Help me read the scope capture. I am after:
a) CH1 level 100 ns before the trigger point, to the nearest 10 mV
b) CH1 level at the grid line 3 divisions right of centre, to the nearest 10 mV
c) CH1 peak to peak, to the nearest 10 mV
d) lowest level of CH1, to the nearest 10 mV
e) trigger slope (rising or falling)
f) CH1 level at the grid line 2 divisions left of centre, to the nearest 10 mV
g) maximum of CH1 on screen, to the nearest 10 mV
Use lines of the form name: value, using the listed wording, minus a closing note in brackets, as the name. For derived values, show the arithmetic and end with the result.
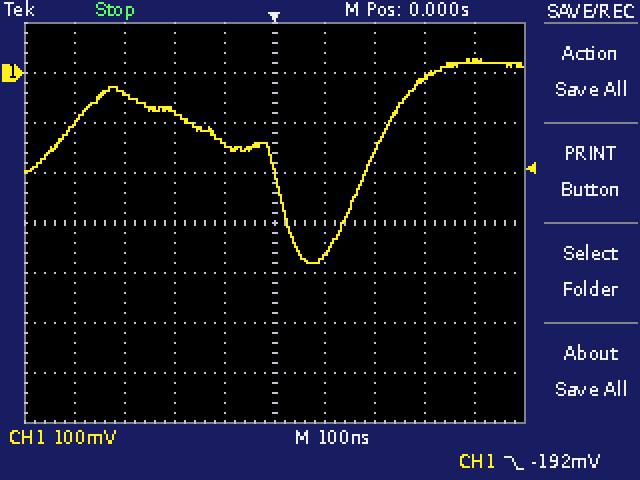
CH1 level 100 ns before the trigger point, to the nearest 10 mV: -140 mV
CH1 level at the grid line 3 divisions right of centre, to the nearest 10 mV: -10 mV
CH1 peak to peak, to the nearest 10 mV: 30 mV − (-380 mV) = 410 mV
lowest level of CH1, to the nearest 10 mV: -380 mV
trigger slope: falling
CH1 level at the grid line 2 divisions left of centre, to the nearest 10 mV: -80 mV
maximum of CH1 on screen, to the nearest 10 mV: 30 mV
